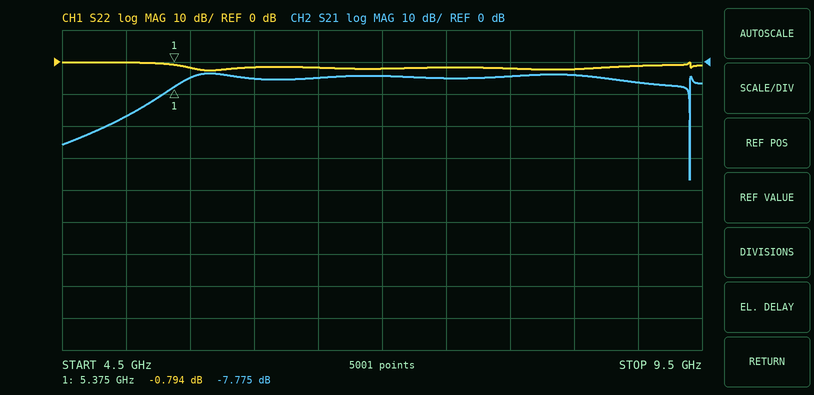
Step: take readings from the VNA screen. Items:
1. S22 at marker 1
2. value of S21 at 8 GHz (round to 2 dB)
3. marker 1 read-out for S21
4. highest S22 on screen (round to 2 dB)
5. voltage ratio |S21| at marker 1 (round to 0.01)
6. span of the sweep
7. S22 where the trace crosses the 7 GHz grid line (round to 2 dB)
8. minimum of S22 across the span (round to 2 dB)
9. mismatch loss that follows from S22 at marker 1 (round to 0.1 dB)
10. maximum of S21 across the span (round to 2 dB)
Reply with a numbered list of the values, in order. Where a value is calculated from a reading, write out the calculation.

1. -0.794 dB
2. -4 dB
3. -7.775 dB
4. 0 dB
5. 10^(-7.775/20) ≈ 0.41
6. 5 GHz
7. -2 dB
8. -2 dB
9. −10 log10(1 − 10^(-0.794/10)) ≈ 7.8 dB
10. -4 dB
